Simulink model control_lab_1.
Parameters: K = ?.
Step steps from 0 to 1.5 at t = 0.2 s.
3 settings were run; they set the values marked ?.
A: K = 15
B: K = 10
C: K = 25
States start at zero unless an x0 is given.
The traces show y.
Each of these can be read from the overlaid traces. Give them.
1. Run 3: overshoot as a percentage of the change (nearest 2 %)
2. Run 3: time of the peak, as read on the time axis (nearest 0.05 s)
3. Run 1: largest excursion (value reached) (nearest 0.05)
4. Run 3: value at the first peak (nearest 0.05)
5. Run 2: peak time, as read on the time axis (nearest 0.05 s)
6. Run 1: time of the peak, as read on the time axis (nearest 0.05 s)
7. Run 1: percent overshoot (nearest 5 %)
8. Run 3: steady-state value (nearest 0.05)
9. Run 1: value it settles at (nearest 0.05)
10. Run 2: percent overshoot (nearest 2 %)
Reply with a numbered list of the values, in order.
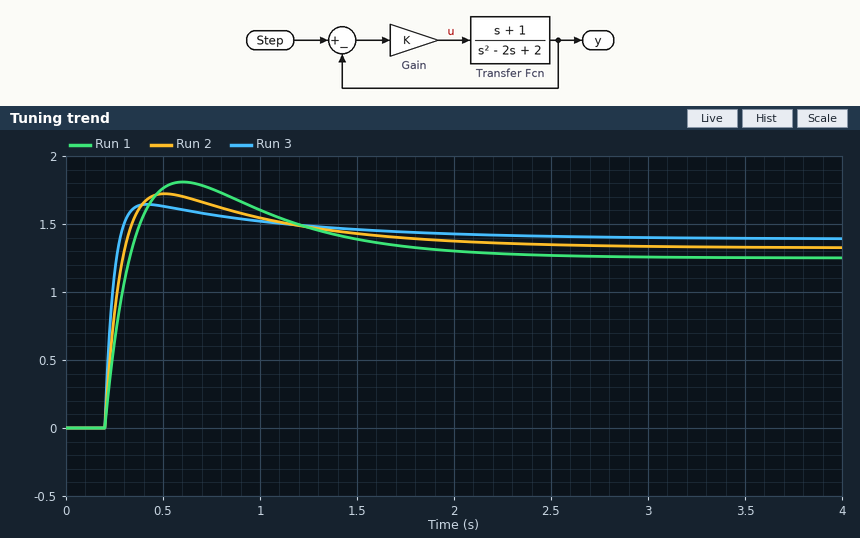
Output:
1. 18 %
2. 0.40 s
3. 1.80
4. 1.65
5. 0.50 s
6. 0.60 s
7. 45 %
8. 1.40
9. 1.25
10. 30 %
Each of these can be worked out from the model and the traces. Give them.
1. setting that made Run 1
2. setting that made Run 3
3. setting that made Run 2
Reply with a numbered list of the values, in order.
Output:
1. B
2. C
3. A
